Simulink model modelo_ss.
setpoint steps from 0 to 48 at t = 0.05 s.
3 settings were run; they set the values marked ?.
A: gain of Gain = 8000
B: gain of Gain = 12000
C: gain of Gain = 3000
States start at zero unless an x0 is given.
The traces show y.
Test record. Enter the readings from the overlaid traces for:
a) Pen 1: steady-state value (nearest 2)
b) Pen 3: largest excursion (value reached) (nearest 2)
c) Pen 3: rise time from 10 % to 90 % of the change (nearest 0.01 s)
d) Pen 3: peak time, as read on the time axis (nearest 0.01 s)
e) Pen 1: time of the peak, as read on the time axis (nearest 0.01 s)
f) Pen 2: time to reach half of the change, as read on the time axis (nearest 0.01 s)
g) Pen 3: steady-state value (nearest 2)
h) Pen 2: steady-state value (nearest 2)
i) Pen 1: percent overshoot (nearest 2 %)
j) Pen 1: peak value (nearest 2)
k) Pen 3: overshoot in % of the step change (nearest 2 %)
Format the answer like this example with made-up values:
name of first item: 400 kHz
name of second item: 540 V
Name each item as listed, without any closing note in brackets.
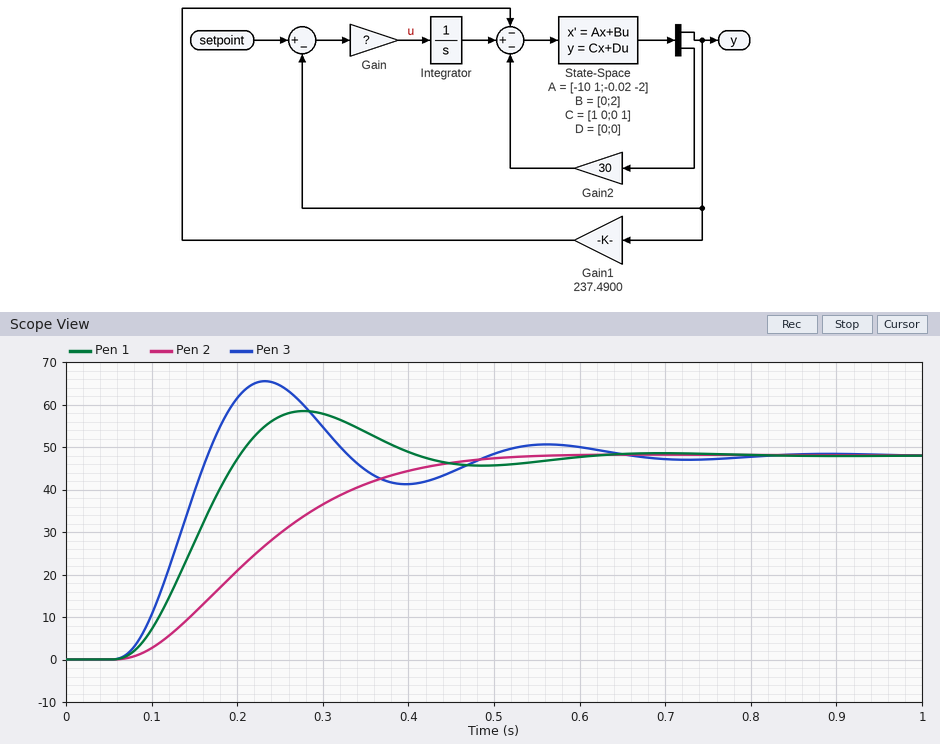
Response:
Pen 1: steady-state value: 48
Pen 3: largest excursion (value reached): 66
Pen 3: rise time from 10 % to 90 % of the change: 0.07 s
Pen 3: peak time, as read on the time axis: 0.23 s
Pen 1: time of the peak, as read on the time axis: 0.28 s
Pen 2: time to reach half of the change, as read on the time axis: 0.22 s
Pen 3: steady-state value: 48
Pen 2: steady-state value: 48
Pen 1: percent overshoot: 22 %
Pen 1: peak value: 58
Pen 3: overshoot in % of the step change: 36 %
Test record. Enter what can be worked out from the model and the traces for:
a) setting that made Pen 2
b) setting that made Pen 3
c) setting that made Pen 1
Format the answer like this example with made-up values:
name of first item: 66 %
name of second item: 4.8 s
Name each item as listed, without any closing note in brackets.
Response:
setting that made Pen 2: C
setting that made Pen 3: B
setting that made Pen 1: A
